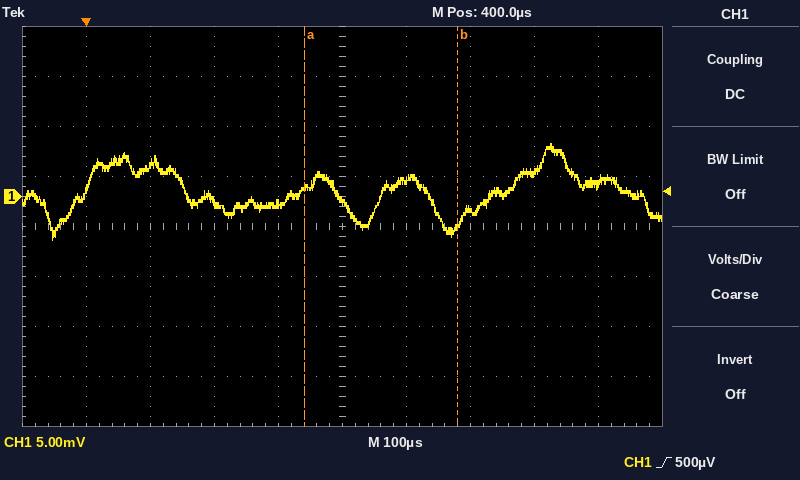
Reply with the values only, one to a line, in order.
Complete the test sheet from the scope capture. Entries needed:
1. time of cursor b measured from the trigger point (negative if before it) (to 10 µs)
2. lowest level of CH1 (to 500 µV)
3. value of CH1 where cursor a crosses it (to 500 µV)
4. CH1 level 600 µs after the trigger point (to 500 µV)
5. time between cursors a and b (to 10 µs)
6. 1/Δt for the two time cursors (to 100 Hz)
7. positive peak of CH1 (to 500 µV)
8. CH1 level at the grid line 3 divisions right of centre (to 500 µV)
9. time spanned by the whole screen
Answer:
+580 µs
-4.5 mV
1.0 mV
-1.5 mV
240 µs
4.2 kHz
5.5 mV
2.5 mV
1 ms
